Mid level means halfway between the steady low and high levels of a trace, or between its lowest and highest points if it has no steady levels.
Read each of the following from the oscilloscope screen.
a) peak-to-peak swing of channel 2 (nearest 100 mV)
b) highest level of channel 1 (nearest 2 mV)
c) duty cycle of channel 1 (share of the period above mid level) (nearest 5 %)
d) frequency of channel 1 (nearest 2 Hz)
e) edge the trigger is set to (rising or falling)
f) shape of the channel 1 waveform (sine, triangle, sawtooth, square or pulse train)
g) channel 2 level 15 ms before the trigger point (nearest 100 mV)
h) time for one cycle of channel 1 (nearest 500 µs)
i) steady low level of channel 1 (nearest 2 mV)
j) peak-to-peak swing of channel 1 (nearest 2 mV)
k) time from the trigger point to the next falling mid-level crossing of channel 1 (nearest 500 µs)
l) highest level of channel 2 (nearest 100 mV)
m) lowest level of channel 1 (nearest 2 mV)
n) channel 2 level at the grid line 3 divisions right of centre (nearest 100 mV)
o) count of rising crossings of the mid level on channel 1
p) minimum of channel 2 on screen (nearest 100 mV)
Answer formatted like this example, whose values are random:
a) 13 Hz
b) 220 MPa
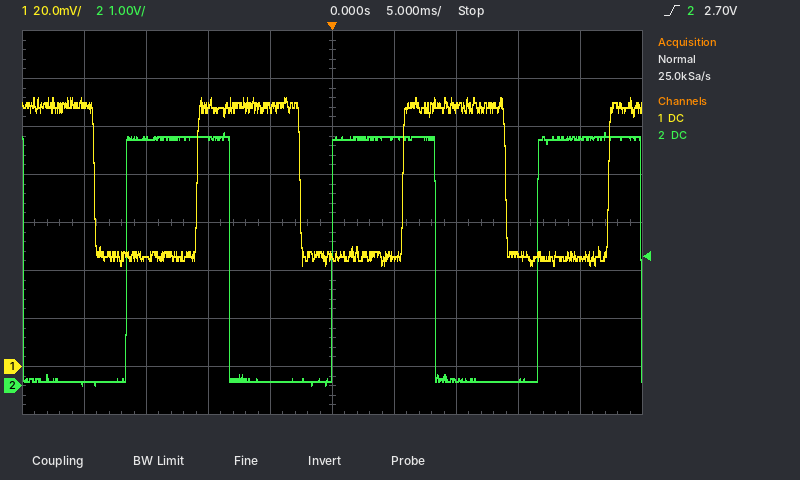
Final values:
a) 5.3 V
b) 112 mV
c) 50 %
d) 60 Hz
e) rising
f) square
g) 5.2 V
h) 16.5 ms
i) 46 mV
j) 70 mV
k) 14.0 ms
l) 5.3 V
m) 42 mV
n) 100 mV
o) 3
p) 0.0 V
